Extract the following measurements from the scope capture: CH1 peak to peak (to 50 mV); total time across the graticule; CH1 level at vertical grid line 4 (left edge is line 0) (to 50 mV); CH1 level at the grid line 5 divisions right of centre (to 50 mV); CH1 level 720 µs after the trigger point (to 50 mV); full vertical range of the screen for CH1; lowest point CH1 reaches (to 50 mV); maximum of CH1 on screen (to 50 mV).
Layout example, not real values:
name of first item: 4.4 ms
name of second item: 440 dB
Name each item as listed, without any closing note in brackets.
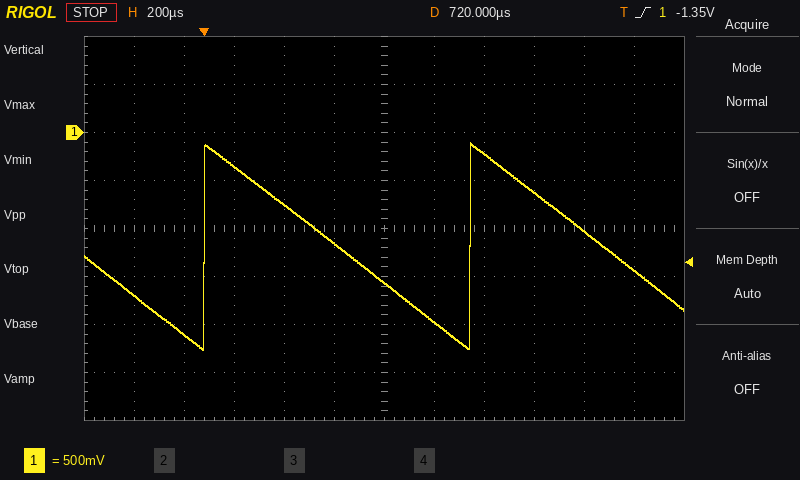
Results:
CH1 peak to peak: 2.15 V
total time across the graticule: 2.4 ms
CH1 level at vertical grid line 4 (left edge is line 0): -750 mV
CH1 level at the grid line 5 divisions right of centre: -1.45 V
CH1 level 720 µs after the trigger point: -1.55 V
full vertical range of the screen for CH1: 4 V
lowest point CH1 reaches: -2.25 V
maximum of CH1 on screen: -100 mV
